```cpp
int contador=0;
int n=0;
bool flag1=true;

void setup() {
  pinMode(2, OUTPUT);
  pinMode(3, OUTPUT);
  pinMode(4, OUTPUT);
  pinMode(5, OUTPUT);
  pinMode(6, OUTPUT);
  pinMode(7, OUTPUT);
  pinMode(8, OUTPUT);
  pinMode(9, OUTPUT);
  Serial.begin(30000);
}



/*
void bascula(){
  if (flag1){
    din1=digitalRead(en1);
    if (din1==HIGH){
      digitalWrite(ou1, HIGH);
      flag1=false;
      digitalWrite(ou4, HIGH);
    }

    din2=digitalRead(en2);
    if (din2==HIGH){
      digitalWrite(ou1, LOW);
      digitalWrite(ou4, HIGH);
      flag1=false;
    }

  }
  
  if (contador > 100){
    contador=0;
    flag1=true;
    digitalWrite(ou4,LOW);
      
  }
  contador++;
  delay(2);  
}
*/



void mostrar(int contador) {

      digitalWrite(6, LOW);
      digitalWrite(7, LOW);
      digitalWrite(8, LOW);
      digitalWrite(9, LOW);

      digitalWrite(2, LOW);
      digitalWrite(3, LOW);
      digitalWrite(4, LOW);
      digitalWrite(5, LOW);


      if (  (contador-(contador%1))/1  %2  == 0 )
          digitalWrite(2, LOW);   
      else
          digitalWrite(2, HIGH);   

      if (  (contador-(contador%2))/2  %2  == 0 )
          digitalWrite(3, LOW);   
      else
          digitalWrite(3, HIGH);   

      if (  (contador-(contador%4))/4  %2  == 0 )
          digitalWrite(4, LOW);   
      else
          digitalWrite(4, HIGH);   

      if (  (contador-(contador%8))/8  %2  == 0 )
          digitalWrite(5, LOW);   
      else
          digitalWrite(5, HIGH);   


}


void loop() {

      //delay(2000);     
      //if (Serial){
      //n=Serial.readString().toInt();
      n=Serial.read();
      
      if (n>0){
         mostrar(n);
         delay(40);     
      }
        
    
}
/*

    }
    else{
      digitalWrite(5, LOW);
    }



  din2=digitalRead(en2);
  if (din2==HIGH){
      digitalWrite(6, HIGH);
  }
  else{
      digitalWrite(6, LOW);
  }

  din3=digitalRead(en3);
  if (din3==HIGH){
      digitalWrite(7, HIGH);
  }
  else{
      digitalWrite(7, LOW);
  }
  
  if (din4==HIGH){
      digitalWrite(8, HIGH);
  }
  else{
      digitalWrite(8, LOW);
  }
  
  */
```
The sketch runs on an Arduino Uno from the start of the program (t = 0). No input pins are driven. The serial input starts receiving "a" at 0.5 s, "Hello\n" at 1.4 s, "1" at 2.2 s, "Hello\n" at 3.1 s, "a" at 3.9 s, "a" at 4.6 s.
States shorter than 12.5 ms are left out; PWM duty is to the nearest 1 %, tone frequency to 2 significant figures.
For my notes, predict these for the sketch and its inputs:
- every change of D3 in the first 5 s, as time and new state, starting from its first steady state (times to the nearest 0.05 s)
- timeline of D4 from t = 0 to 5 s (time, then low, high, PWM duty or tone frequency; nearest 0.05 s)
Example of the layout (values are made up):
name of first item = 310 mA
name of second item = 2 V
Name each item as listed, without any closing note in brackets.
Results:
every change of D3 in the first 5 s, as time and new state, starting from its first steady state = 0 s low; 1.55 s high; 2.2 s low; 3.25 s high; 3.9 s low
timeline of D4 from t = 0 to 5 s = 0 s low; 1.45 s high; 1.6 s low; 3.15 s high; 3.3 s low
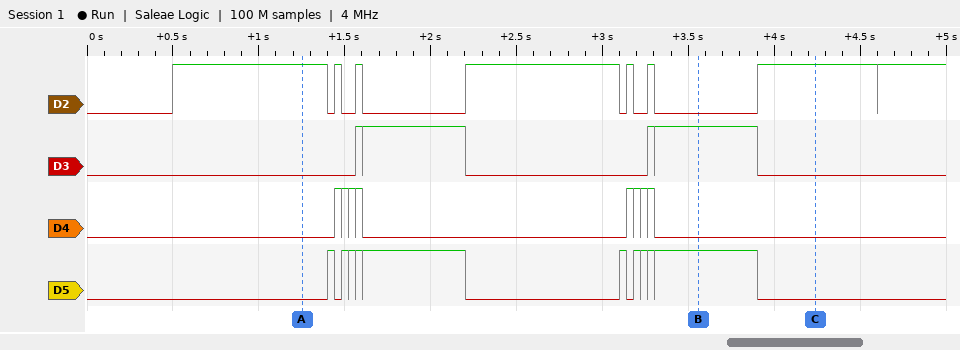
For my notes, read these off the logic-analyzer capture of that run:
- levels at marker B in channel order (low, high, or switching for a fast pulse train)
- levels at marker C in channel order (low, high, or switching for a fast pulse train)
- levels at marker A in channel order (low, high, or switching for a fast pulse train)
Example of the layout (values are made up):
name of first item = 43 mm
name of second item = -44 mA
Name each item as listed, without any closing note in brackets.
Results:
levels at marker B in channel order = D2 low, D3 high, D4 low, D5 high
levels at marker C in channel order = D2 high, D3 low, D4 low, D5 low
levels at marker A in channel order = D2 high, D3 low, D4 low, D5 low
